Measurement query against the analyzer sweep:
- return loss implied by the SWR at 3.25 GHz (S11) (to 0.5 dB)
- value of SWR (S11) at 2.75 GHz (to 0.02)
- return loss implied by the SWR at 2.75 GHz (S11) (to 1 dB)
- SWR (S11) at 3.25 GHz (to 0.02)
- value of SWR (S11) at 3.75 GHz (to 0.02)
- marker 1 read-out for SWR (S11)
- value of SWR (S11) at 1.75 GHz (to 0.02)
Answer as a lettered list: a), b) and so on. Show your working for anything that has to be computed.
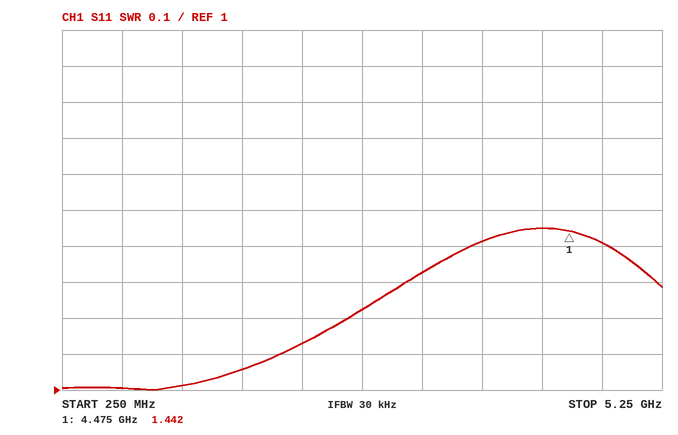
a) −20 log10((1.32 − 1)/(1.32 + 1)) ≈ 17.2 dB, so 17.0 dB to the nearest 0.5 dB
b) 1.22
c) −20 log10((1.22 − 1)/(1.22 + 1)) ≈ 20 dB
d) 1.32
e) 1.42
f) 1.442
g) 1.06
